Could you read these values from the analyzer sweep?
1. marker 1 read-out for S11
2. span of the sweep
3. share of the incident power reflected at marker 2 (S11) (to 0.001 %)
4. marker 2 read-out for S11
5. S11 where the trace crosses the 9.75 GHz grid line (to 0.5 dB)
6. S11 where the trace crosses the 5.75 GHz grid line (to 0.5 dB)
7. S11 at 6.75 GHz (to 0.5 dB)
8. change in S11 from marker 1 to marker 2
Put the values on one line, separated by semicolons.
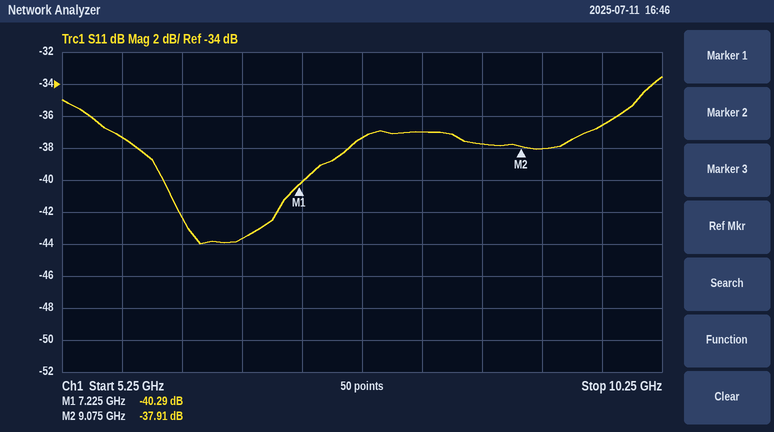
-40.29 dB; 5 GHz; 0.016 %; -37.91 dB; -36.5 dB; -37.5 dB; -43.5 dB; 2.38 dB
